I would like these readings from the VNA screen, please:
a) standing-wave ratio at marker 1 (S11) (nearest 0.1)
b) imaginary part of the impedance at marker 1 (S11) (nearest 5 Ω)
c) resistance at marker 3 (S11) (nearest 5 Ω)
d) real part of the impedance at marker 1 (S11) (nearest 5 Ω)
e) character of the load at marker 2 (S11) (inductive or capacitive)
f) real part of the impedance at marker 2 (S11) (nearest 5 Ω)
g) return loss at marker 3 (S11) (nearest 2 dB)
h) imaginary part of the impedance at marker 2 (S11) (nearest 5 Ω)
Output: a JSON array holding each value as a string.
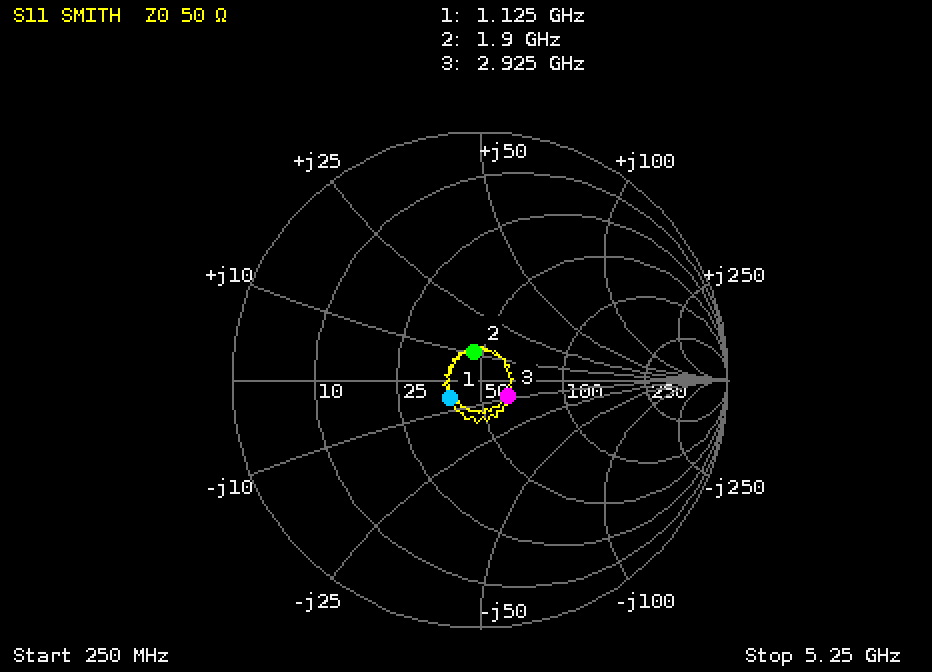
["1.3", "-5 Ω", "60 Ω", "40 Ω", "inductive", "45 Ω", "18 dB", "+10 Ω"]
